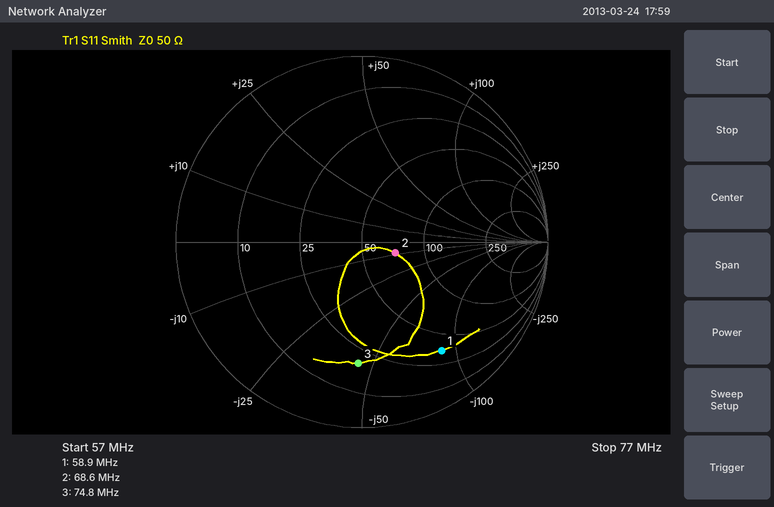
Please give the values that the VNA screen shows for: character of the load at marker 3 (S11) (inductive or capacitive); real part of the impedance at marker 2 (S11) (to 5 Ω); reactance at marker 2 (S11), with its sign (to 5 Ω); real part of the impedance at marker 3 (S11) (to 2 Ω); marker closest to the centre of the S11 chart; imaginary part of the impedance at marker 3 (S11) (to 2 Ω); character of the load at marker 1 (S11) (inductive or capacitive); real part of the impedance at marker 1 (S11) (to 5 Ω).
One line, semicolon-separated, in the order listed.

capacitive; 70 Ω; -10 Ω; 20 Ω; marker 2; -44 Ω; capacitive; 35 Ω
